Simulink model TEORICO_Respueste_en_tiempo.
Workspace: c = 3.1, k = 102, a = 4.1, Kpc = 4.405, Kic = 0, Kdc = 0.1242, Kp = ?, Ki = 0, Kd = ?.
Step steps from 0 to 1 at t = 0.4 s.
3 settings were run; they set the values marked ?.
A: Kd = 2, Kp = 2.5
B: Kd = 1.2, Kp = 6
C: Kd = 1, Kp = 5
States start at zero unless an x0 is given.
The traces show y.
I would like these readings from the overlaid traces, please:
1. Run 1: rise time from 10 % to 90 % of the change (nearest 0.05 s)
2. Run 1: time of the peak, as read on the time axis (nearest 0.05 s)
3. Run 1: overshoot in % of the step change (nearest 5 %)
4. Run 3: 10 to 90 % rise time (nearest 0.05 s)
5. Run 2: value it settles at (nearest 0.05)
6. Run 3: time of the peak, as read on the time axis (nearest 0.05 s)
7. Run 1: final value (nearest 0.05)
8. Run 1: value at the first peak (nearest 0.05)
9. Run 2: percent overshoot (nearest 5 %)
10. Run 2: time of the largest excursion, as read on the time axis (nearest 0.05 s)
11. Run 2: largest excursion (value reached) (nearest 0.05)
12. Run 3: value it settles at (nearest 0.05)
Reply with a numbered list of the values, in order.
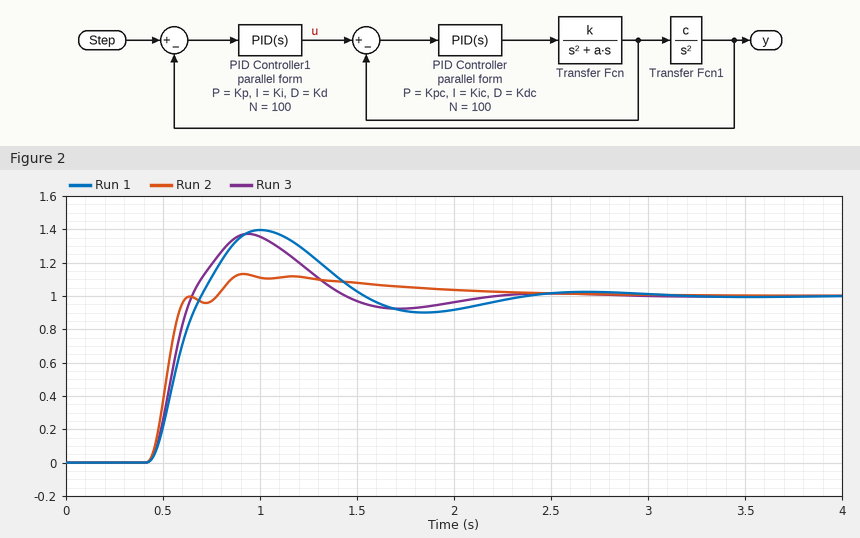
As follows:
1. 0.20 s
2. 1.00 s
3. 40 %
4. 0.15 s
5. 1.00
6. 0.95 s
7. 1.00
8. 1.40
9. 15 %
10. 0.90 s
11. 1.15
12. 1.00
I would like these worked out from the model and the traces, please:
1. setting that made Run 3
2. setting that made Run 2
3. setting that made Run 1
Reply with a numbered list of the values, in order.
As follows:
1. B
2. A
3. C
